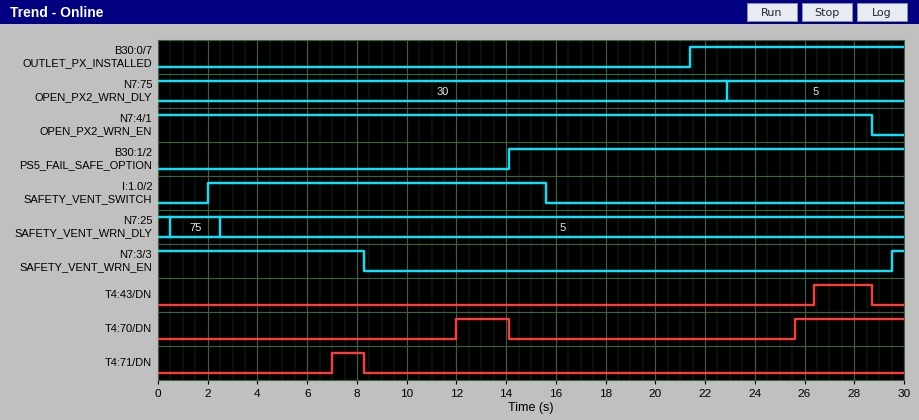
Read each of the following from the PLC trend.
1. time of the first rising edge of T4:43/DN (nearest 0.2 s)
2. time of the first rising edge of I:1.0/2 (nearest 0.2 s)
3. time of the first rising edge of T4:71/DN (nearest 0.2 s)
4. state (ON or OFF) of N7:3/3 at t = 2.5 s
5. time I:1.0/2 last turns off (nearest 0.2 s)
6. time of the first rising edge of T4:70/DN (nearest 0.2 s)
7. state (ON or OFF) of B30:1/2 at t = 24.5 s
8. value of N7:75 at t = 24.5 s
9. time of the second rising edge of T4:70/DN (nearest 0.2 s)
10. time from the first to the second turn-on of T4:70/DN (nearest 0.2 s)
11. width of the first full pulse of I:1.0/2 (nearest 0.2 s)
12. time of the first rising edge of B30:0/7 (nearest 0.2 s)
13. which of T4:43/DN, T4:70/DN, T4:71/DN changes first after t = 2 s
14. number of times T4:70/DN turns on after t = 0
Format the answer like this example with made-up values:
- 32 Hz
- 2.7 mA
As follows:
- 26.4 s
- 2.0 s
- 7.0 s
- ON
- 15.6 s
- 12.0 s
- ON
- 5
- 25.6 s
- 13.6 s
- 13.6 s
- 21.4 s
- T4:71/DN
- 2
